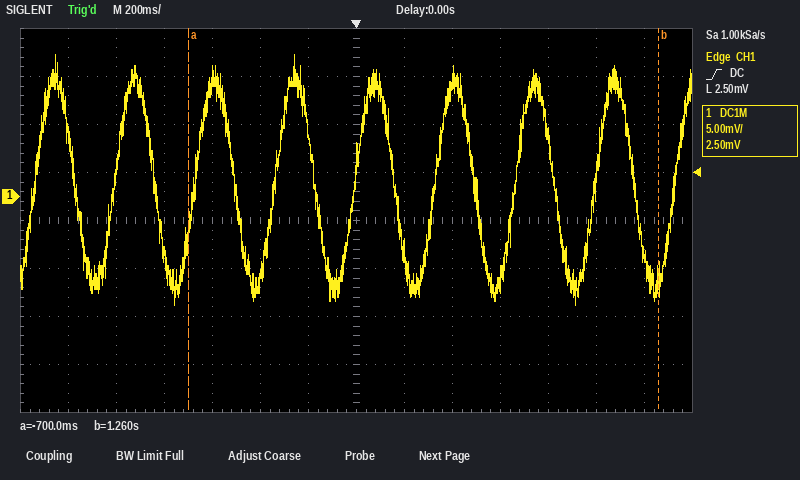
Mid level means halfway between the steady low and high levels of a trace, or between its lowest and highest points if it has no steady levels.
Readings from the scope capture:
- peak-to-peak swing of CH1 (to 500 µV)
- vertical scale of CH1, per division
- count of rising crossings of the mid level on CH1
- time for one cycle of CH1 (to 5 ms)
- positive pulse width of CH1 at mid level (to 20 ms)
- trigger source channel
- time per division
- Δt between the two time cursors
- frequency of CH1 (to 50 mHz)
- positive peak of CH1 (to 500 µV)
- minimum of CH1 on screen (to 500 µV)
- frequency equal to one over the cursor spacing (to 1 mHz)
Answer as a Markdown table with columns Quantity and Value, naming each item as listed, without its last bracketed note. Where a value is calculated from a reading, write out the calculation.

| Quantity | Value |
|---|---|
| peak-to-peak swing of CH1 | 15.0 mV − (-11.0 mV) = 26.0 mV |
| vertical scale of CH1, per division | 5 mV |
| count of rising crossings of the mid level on CH1 | 9 |
| time for one cycle of CH1 | 335 ms |
| positive pulse width of CH1 at mid level | 160 ms |
| trigger source channel | CH1 |
| time per division | 200 ms |
| Δt between the two time cursors | 1.26 s − (-700 ms) = 1.96 s |
| frequency of CH1 | 1 / 335 ms ≈ 2.99 Hz, so 3.00 Hz to the nearest 50 mHz |
| positive peak of CH1 | 15.0 mV |
| minimum of CH1 on screen | -11.0 mV |
| frequency equal to one over the cursor spacing | 1 / 1.96 s ≈ 510 mHz |
